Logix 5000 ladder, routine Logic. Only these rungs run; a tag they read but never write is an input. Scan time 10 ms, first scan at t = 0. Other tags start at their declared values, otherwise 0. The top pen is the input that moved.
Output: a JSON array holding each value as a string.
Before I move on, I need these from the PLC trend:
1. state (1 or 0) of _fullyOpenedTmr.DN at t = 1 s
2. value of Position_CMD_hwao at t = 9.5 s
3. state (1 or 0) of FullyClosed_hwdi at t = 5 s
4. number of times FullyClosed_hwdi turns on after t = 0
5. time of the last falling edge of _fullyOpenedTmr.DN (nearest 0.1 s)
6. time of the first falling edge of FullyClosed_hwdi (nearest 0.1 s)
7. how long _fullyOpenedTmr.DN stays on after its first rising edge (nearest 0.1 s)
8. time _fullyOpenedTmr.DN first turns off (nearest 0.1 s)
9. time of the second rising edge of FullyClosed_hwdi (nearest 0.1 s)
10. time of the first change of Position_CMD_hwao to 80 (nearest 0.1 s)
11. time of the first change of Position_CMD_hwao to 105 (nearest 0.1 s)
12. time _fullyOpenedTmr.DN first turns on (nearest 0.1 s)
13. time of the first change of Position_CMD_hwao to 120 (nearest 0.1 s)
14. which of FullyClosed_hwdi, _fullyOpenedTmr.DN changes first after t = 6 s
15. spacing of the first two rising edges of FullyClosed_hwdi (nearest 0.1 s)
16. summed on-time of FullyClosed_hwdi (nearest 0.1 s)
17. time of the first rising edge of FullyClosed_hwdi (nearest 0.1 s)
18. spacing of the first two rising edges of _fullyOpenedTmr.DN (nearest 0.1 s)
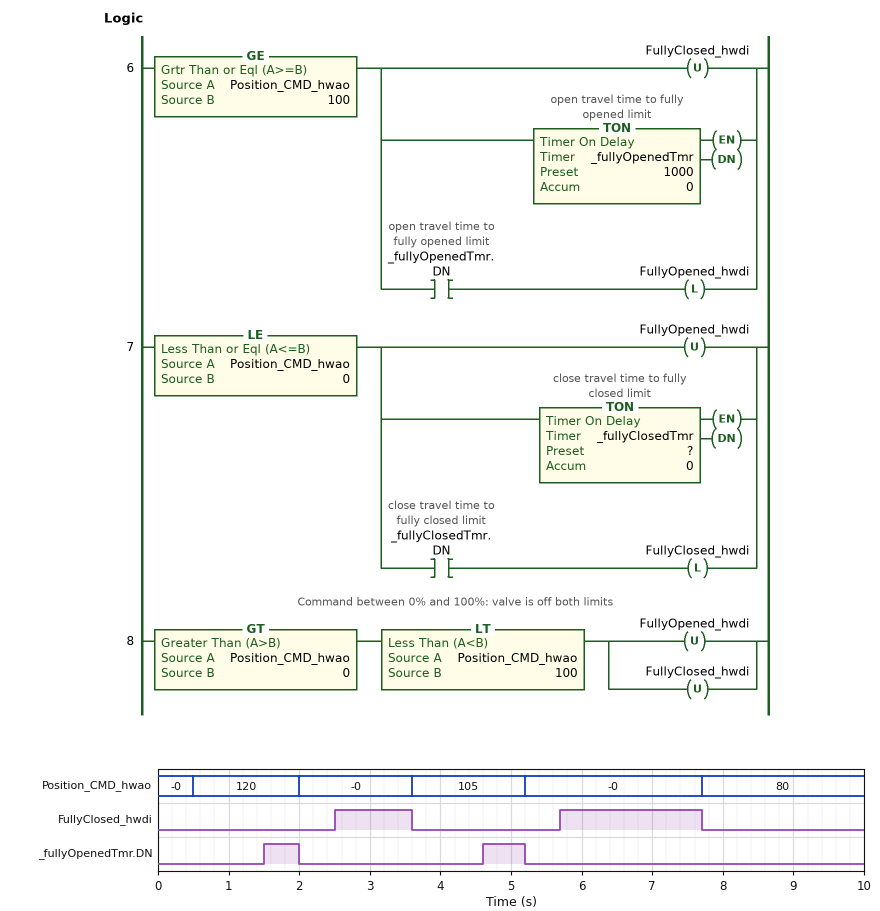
["0", "80", "0", "2", "5.2 s", "3.6 s", "0.5 s", "2.0 s", "5.7 s", "7.7 s", "3.6 s", "1.5 s", "0.5 s", "FullyClosed_hwdi", "3.2 s", "3.1 s", "2.5 s", "3.1 s"]
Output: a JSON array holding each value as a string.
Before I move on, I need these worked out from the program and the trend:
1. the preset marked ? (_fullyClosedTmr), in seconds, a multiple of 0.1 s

["0.5 s"]
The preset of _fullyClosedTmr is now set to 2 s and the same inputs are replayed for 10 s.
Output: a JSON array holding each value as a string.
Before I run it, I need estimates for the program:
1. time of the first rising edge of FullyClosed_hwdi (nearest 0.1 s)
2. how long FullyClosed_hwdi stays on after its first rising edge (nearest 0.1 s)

["7.2 s", "0.5 s"]
